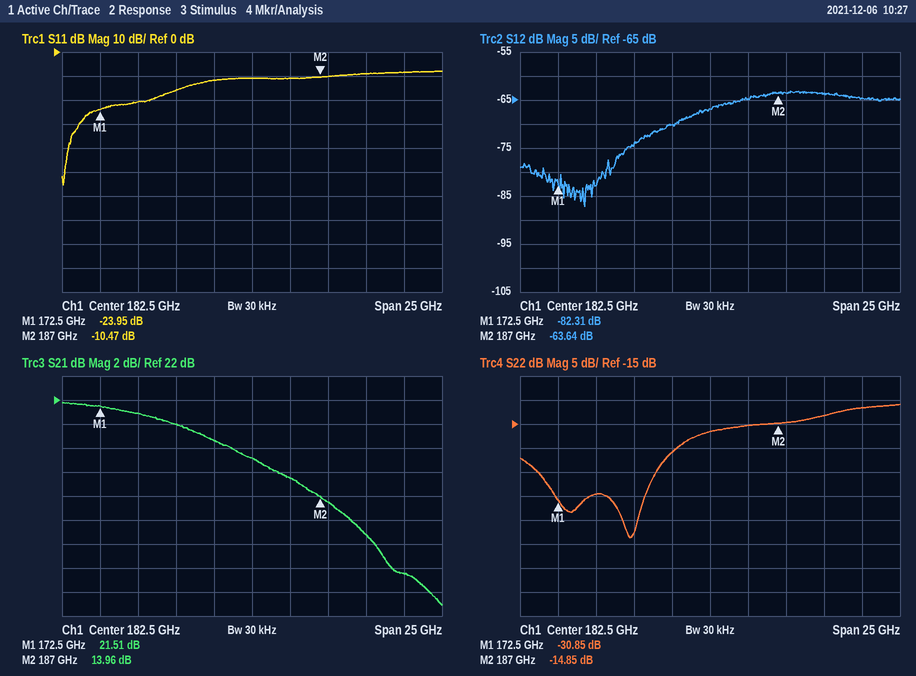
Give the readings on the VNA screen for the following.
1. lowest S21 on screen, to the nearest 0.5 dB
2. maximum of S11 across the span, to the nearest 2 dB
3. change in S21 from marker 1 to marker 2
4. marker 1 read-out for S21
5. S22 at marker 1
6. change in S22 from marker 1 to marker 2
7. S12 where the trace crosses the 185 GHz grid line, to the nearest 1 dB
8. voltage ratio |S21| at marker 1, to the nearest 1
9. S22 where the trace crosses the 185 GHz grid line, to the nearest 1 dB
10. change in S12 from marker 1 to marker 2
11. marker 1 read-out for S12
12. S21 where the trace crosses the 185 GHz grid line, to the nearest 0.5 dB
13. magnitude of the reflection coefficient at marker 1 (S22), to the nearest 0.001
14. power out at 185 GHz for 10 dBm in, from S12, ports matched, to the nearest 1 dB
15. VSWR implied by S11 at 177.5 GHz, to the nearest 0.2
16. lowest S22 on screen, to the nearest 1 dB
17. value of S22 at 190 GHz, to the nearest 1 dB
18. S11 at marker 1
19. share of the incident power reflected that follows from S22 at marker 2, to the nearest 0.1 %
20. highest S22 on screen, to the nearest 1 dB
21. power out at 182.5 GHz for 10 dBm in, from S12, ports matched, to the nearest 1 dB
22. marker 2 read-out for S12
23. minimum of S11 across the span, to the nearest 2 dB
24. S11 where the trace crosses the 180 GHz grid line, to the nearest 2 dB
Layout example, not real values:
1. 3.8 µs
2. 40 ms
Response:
1. 5.0 dB
2. -8 dB
3. -7.55 dB
4. 21.51 dB
5. -30.85 dB
6. 16.00 dB
7. -65 dB
8. 12
9. -15 dB
10. 18.67 dB
11. -82.31 dB
12. 15.5 dB
13. 0.029
14. -55 dBm
15. 1.4
16. -39 dB
17. -13 dB
18. -23.95 dB
19. 3.3 %
20. -11 dB
21. -57 dBm
22. -63.64 dB
23. -56 dB
24. -12 dB
